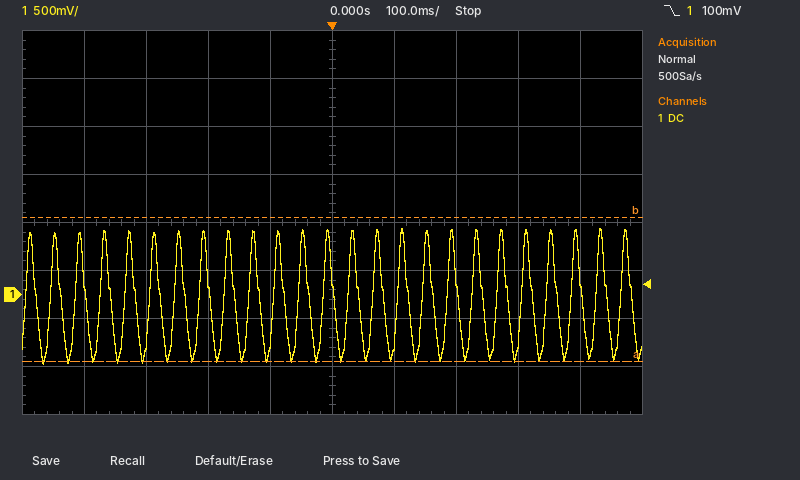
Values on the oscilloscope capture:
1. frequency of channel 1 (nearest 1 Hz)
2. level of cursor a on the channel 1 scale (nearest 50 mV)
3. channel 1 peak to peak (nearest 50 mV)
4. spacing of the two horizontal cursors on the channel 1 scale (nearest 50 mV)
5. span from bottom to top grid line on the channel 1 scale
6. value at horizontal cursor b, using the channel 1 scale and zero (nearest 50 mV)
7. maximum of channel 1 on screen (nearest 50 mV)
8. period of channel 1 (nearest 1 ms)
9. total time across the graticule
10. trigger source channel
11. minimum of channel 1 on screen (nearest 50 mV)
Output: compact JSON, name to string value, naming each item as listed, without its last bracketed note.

{"frequency of channel 1": "25 Hz", "level of cursor a on the channel 1 scale": "-700 mV", "channel 1 peak to peak": "1.40 V", "spacing of the two horizontal cursors on the channel 1 scale": "1.50 V", "span from bottom to top grid line on the channel 1 scale": "4 V", "value at horizontal cursor b, using the channel 1 scale and zero": "800 mV", "maximum of channel 1 on screen": "700 mV", "period of channel 1": "40 ms", "total time across the graticule": "1 s", "trigger source channel": "channel 1", "minimum of channel 1 on screen": "-700 mV"}
